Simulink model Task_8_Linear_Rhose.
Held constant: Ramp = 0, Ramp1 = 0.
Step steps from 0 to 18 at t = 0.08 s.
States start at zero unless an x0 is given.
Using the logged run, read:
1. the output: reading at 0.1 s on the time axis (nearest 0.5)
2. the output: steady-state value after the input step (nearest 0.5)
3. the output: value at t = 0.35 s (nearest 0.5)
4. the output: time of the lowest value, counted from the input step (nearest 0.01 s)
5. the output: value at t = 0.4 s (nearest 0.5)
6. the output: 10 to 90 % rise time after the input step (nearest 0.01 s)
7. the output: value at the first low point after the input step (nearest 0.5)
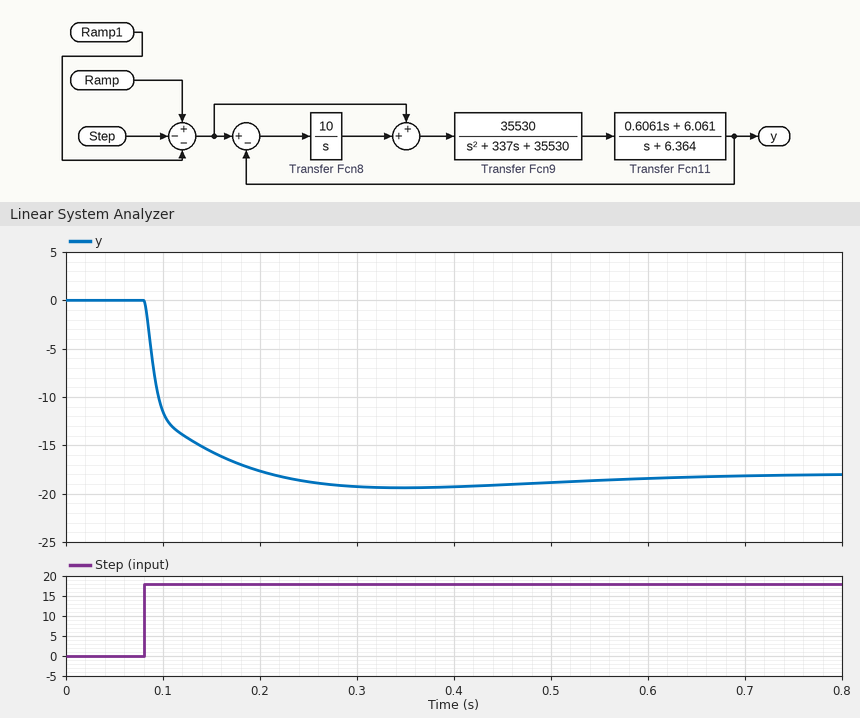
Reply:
-11.5
-18.0
-19.5
0.27 s
-19.5
0.08 s
-19.5
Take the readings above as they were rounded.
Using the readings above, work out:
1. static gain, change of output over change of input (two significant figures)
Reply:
-1.0
